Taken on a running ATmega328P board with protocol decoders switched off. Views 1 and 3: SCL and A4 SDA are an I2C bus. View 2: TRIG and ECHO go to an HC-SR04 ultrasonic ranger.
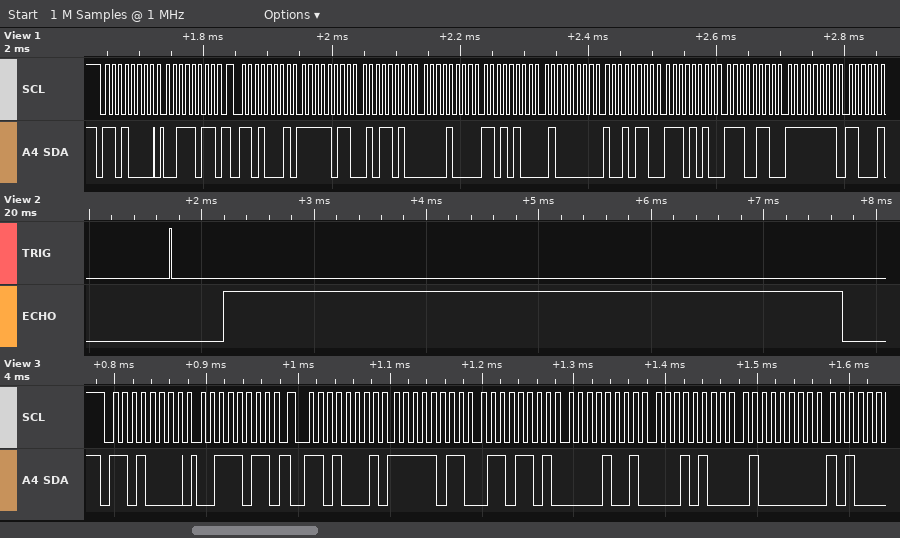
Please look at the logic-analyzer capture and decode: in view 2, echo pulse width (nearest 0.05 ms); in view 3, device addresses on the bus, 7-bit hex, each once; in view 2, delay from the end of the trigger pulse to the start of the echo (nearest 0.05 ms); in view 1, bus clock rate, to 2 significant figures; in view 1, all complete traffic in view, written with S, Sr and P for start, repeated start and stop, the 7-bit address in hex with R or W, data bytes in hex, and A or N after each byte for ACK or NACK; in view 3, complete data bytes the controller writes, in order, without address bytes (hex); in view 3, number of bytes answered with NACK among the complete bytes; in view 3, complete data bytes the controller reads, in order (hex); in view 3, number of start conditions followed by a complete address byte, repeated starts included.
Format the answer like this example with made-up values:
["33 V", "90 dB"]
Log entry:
["5.50 ms", "0x68", "0.45 ms", "100 kHz", "S 68W A 3B A Sr 68R A FB A 5A A 08 A D4 A 40 A 96 A EA A E6 A FF A", "3B", "0", "FB 6D 09 14 40", "2"]
